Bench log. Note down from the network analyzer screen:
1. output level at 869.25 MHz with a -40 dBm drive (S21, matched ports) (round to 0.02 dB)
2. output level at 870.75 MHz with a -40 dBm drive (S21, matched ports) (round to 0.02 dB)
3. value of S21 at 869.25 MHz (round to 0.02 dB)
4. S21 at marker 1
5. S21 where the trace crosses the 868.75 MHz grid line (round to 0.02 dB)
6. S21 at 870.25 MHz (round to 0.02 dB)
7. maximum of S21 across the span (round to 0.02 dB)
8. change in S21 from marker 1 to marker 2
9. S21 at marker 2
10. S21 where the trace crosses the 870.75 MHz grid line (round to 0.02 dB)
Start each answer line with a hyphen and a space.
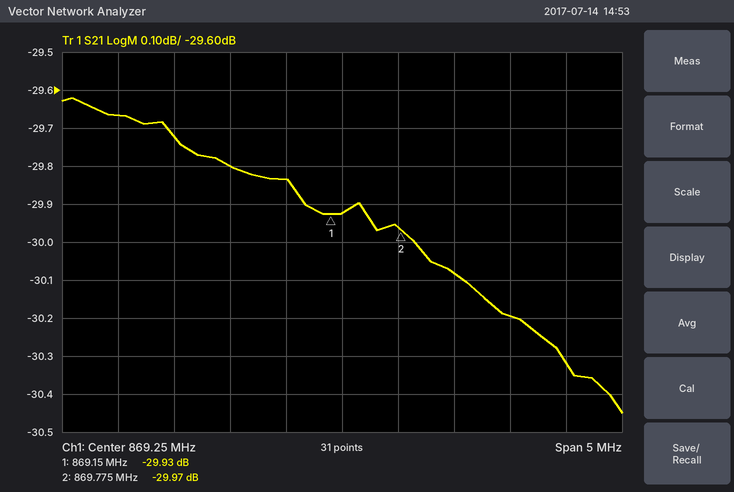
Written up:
- -69.92 dBm
- -70.20 dBm
- -29.92 dB
- -29.93 dB
- -29.84 dB
- -30.08 dB
- -29.62 dB
- -0.04 dB
- -29.97 dB
- -30.20 dB
